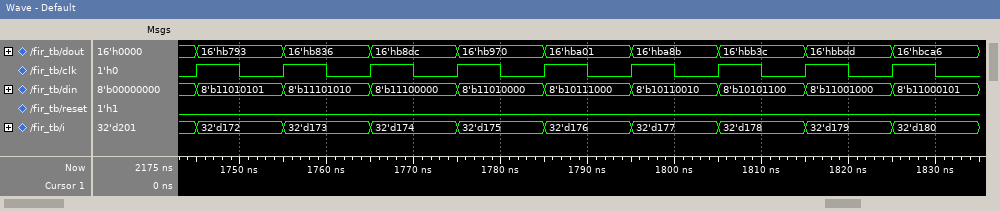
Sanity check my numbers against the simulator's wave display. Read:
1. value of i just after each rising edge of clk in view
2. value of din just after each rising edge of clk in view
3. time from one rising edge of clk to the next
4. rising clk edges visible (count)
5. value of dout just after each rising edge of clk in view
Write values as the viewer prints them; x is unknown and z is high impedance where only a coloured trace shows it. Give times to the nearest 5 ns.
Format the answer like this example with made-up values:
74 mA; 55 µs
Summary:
32'd172, 32'd173, 32'd174, 32'd175, 32'd176, 32'd177, 32'd178, 32'd179, 32'd180; 8'b11010101, 8'b11101010, 8'b11100000, 8'b11010000, 8'b10111000, 8'b10110010, 8'b10101100, 8'b11001000, 8'b11000101; 10 ns; 9; 16'hb793, 16'hb836, 16'hb8dc, 16'hb970, 16'hba01, 16'hba8b, 16'hbb3c, 16'hbbdd, 16'hbca6
